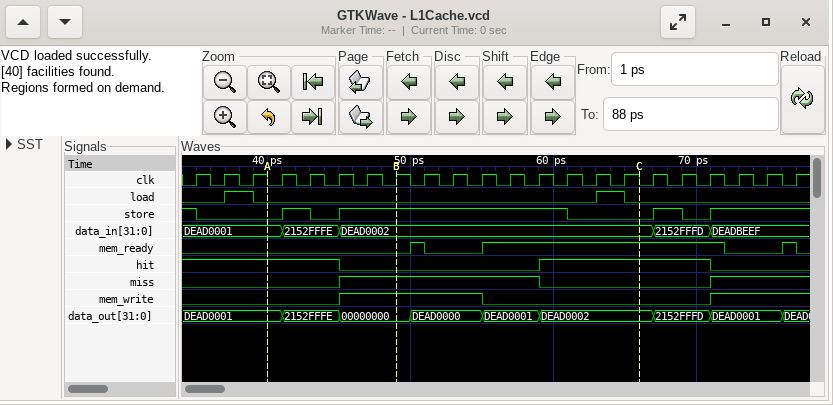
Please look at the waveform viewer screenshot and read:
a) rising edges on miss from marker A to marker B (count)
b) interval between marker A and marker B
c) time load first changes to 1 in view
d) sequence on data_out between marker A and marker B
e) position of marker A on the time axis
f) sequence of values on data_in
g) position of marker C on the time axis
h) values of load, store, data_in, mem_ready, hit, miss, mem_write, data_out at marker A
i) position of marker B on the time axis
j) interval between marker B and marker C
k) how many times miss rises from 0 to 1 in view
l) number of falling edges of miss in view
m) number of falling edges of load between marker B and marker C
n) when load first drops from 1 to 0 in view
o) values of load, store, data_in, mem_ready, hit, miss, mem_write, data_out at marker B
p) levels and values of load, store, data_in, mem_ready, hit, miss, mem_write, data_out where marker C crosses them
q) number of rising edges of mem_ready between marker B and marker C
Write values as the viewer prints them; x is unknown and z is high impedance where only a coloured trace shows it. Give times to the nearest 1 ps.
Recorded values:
1
9 ps
37 ps
DEAD0001, 2152FFFE, 00000000
40 ps
DEAD0001, 2152FFFE, DEAD0002, 2152FFFD, DEADBEEF
66 ps
load=0, store=0, data_in=DEAD0001, mem_ready=0, hit=1, miss=0, mem_write=0, data_out=DEAD0001
49 ps
17 ps
2
1
1
39 ps
load=0, store=1, data_in=DEAD0002, mem_ready=0, hit=0, miss=1, mem_write=1, data_out=00000000
load=0, store=0, data_in=DEAD0002, mem_ready=1, hit=1, miss=0, mem_write=0, data_out=DEAD0002
2
